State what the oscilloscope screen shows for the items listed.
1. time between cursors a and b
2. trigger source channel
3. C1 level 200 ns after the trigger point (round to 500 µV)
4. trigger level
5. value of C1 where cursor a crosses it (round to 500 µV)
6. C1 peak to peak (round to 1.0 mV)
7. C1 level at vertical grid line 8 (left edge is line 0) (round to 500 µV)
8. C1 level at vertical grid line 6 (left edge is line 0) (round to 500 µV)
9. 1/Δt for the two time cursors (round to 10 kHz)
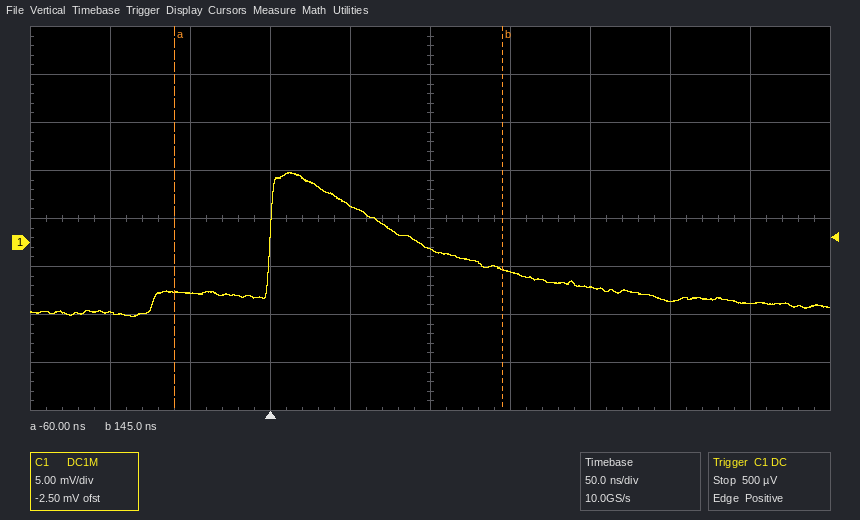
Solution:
205 ns
C1
-4.5 mV
500 µV
-5.0 mV
15.0 mV
-6.0 mV
-3.0 mV
4.88 MHz
